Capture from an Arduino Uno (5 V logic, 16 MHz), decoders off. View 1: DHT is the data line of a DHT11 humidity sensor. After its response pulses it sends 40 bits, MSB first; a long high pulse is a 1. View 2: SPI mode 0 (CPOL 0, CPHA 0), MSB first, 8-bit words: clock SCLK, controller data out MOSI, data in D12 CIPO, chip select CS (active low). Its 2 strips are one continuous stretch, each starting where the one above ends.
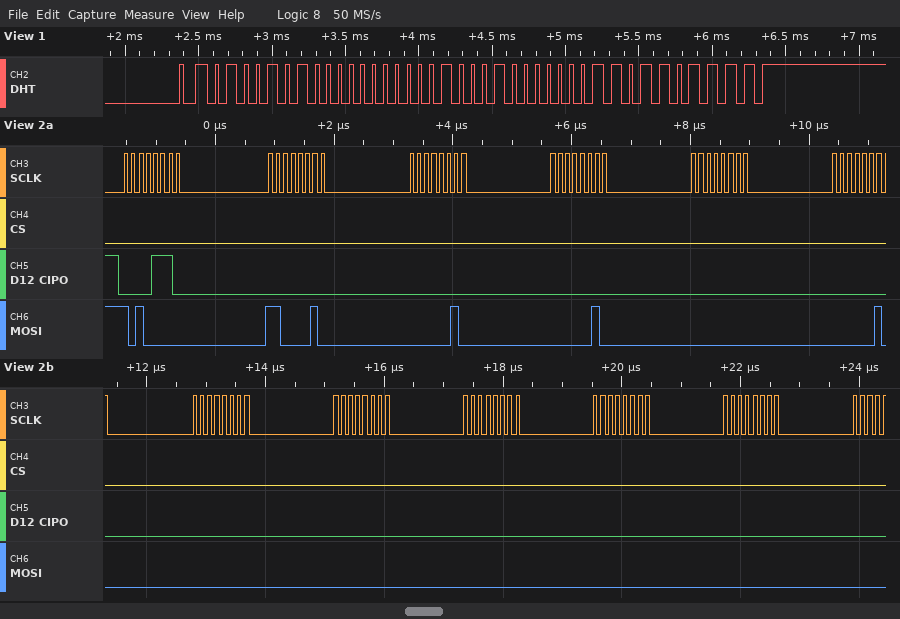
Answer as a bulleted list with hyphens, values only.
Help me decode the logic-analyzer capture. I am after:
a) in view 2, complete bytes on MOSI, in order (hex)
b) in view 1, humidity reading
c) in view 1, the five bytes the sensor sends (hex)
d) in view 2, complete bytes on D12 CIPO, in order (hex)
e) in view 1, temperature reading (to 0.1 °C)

- A0 C2 02 02 00 02 00 00 00 00 00
- 74 %
- 4A 00 22 03 6F
- 0E 00 00 00 00 00 00 00 00 00 00
- 34.3 °C
